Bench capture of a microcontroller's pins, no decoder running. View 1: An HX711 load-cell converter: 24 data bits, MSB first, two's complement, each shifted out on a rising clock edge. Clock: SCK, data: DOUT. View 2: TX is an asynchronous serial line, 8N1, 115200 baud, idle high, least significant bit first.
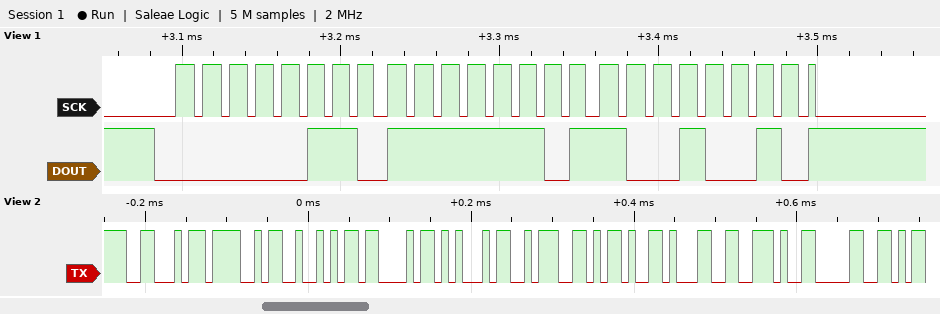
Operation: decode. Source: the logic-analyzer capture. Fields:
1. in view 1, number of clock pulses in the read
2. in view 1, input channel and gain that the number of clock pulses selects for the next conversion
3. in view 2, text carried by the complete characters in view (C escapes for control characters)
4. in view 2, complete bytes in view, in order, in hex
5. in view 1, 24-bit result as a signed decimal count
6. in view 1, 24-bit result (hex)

25
channel A, gain 128
"FORCE:-1.0"
46 4F 52 43 45 3A 2D 31 2E 30
458130
0x06FD92
